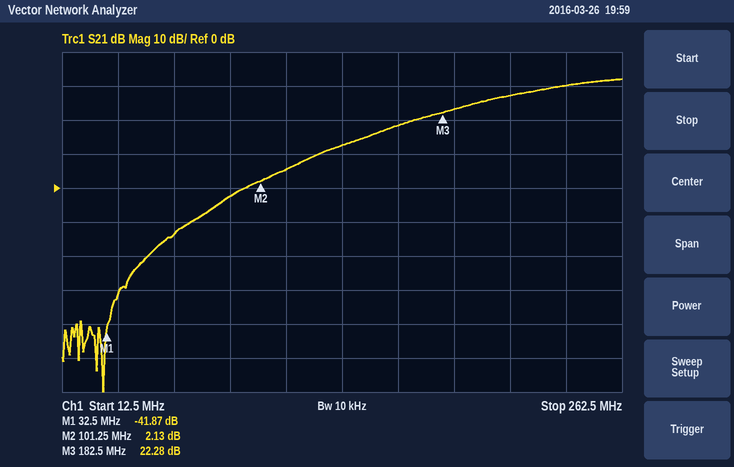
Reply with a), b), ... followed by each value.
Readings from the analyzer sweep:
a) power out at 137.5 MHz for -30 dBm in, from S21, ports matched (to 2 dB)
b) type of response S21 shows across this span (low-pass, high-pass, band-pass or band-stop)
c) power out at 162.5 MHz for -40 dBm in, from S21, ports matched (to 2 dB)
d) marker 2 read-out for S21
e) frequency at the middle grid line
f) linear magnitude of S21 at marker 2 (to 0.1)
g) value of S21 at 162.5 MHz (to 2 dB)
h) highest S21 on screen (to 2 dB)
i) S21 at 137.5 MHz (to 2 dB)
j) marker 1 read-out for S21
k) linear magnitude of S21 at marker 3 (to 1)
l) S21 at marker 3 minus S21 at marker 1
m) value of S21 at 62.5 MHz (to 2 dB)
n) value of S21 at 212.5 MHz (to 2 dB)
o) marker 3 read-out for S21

a) -18 dBm
b) high-pass
c) -22 dBm
d) 2.13 dB
e) 137.5 MHz
f) 1.3
g) 18 dB
h) 32 dB
i) 12 dB
j) -41.87 dB
k) 13
l) 64.15 dB
m) -14 dB
n) 28 dB
o) 22.28 dB
